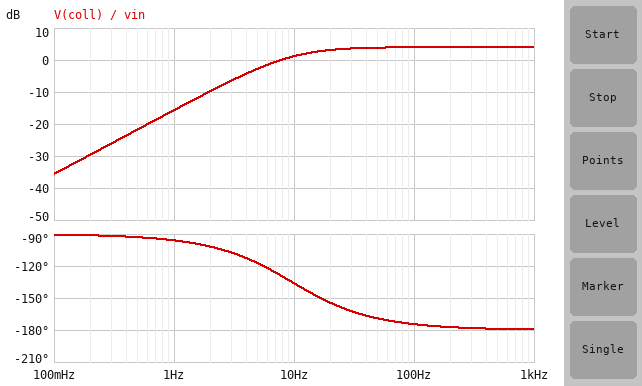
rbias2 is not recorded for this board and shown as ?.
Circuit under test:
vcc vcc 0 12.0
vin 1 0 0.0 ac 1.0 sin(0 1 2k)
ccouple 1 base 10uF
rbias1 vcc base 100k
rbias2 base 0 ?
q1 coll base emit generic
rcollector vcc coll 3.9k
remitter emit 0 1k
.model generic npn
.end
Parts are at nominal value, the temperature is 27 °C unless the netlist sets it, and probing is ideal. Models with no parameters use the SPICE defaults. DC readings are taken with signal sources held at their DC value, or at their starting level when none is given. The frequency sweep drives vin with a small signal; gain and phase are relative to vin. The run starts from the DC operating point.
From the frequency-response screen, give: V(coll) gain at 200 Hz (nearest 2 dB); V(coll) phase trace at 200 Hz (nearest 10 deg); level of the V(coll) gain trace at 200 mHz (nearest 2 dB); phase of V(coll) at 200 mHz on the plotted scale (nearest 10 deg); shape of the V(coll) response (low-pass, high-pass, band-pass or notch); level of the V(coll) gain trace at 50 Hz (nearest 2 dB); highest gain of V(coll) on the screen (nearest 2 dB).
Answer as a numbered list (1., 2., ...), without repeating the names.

1. 4 dB
2. -180 deg
3. -30 dB
4. -90 deg
5. high-pass
6. 4 dB
7. 4 dB
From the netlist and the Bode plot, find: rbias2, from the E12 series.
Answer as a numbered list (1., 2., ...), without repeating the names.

1. 56 kΩ
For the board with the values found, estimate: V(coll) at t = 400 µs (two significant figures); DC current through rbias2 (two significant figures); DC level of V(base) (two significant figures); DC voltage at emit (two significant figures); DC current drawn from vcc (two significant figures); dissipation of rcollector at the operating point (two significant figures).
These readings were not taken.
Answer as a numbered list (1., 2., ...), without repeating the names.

1. 6.3 V
2. 58 µA
3. 3.2 V
4. 2.4 V
5. 2.5 mA
6. 23 mW
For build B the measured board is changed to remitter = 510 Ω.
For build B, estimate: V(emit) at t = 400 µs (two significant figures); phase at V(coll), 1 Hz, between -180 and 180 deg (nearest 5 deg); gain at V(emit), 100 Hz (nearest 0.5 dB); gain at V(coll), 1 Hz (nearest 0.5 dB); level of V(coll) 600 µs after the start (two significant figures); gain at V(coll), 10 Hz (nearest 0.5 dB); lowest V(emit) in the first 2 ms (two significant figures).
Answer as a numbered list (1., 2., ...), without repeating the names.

1. 450 mV
2. -90 deg
3. -0.5 dB
4. -36.0 dB
5. 2.3 V
6. -16.5 dB
7. 320 mV
